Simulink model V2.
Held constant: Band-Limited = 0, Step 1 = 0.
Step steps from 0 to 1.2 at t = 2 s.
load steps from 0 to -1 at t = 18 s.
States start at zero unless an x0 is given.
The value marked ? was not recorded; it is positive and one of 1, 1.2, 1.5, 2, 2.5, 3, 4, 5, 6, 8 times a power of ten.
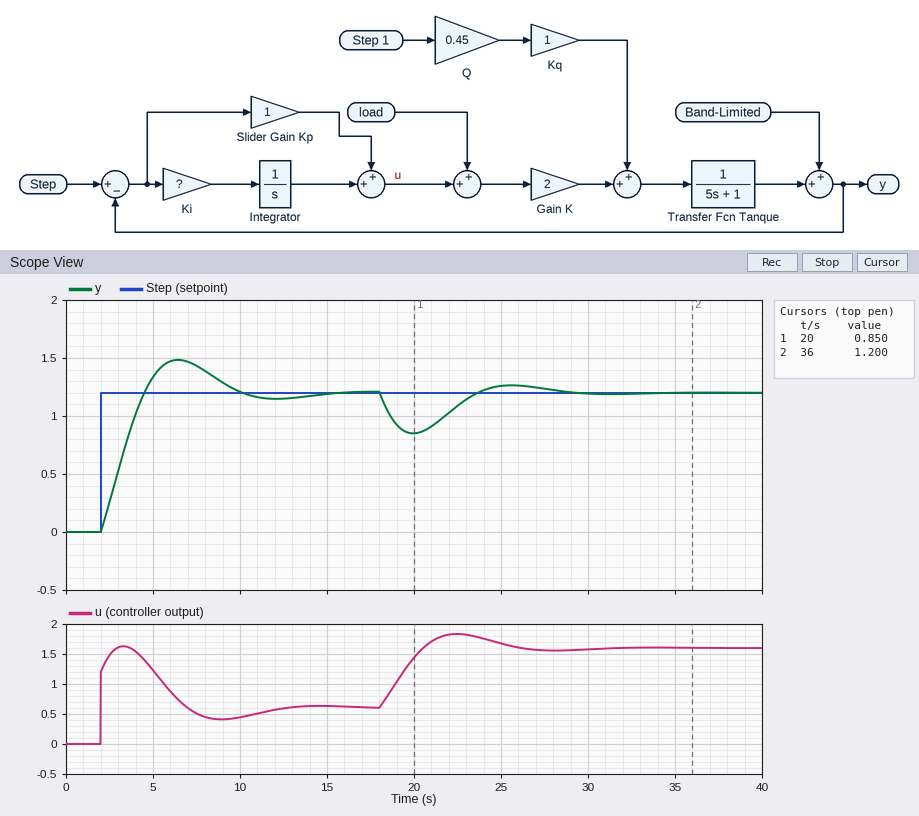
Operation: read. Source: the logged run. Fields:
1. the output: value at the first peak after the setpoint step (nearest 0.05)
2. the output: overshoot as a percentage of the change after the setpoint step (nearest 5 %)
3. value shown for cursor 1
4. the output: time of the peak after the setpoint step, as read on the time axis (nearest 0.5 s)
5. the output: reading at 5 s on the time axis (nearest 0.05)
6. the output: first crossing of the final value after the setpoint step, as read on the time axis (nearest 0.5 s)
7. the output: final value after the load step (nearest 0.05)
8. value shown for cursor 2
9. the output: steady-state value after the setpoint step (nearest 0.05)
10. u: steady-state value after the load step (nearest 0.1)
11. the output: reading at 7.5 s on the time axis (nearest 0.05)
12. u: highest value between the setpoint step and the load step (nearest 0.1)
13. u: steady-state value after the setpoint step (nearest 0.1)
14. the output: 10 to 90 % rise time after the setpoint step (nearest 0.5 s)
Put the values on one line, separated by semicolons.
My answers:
1.50; 25 %; 0.850; 6.5 s; 1.35; 4.5 s; 1.20; 1.200; 1.20; 1.6; 1.45; 1.6; 0.6; 2.0 s
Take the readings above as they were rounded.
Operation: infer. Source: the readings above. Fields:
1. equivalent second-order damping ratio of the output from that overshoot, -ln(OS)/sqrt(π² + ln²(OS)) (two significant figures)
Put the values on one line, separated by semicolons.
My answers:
0.40
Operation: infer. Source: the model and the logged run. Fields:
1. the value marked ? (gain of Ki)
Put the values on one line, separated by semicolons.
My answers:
1
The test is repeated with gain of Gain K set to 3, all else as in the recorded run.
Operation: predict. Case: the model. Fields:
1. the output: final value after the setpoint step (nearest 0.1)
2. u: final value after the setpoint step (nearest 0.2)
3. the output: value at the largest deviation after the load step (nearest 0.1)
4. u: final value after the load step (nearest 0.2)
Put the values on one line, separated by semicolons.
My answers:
1.2; 0.4; 0.8; 1.4
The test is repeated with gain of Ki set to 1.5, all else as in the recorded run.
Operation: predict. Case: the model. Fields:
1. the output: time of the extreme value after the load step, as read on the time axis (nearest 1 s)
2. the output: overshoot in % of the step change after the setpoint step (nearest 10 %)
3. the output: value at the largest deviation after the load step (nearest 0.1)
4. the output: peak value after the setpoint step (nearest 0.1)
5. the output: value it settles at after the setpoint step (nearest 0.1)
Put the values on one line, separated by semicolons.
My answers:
20 s; 30 %; 0.9; 1.6; 1.2
